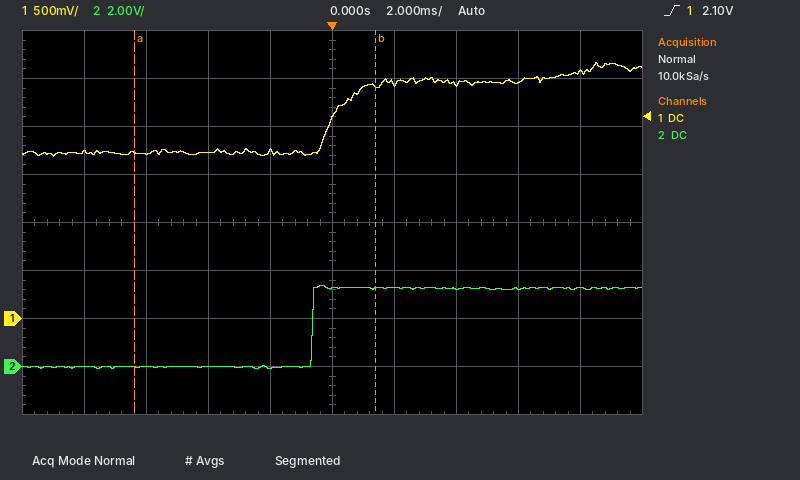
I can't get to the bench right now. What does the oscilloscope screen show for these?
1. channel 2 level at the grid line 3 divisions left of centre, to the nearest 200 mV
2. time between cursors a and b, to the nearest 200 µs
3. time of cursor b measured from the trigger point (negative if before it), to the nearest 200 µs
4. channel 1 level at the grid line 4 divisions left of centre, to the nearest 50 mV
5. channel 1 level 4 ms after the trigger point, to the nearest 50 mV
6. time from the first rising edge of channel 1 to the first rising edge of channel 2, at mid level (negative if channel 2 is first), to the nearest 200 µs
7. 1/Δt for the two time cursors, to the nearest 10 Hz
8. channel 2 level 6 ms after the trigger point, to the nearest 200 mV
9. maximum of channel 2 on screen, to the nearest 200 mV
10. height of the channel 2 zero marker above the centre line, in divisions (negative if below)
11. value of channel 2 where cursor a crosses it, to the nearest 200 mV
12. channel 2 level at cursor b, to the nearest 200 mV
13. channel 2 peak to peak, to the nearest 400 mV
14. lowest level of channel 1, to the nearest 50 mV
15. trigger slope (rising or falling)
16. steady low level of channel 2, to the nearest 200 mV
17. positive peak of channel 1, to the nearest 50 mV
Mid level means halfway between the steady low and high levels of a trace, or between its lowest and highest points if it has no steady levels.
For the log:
0.0 V
7.8 ms
+1.4 ms
1.75 V
2.45 V
-800 µs
130 Hz
3.2 V
3.4 V
-3.0 div
0.0 V
3.2 V
3.6 V
1.70 V
rising
0.0 V
2.65 V
